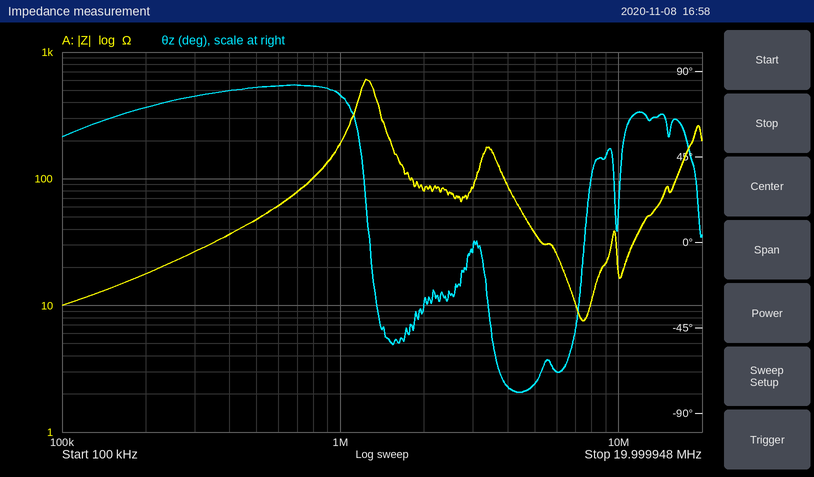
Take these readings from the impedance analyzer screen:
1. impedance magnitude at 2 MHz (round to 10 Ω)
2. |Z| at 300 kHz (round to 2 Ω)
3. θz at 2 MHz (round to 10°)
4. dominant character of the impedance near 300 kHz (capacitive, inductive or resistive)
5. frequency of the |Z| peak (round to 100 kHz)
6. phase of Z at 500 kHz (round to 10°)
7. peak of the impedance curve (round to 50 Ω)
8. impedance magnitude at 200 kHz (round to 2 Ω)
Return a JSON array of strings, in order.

["80 Ω", "26 Ω", "-30°", "inductive", "1.2 MHz", "80°", "600 Ω", "18 Ω"]
